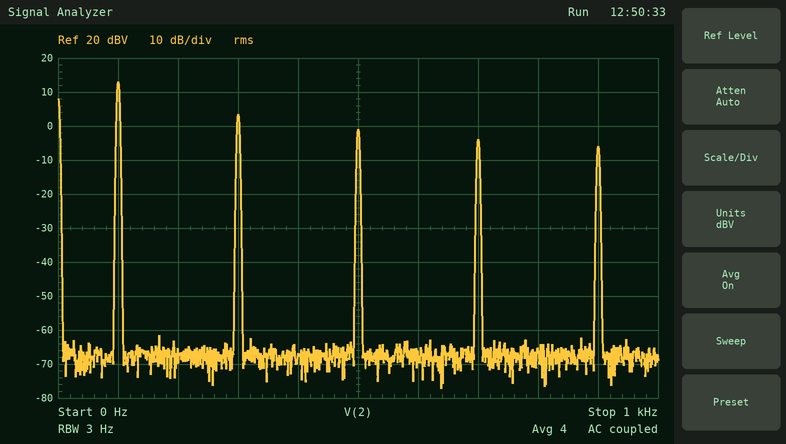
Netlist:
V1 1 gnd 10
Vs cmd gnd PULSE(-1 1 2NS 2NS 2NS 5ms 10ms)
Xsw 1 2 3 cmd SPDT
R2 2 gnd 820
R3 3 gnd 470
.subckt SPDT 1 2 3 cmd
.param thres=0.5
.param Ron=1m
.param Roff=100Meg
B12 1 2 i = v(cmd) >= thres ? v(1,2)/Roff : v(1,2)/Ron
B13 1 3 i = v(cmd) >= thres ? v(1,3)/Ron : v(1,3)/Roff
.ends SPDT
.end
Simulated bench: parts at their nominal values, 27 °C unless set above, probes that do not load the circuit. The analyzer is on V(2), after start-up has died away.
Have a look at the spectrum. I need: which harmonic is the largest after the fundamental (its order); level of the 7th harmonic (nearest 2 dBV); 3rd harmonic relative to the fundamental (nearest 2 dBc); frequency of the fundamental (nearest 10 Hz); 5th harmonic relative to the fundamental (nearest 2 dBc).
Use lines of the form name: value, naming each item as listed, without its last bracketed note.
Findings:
which harmonic is the largest after the fundamental: 3
level of the 7th harmonic: -4 dBV
3rd harmonic relative to the fundamental: -10 dBc
frequency of the fundamental: 100 Hz
5th harmonic relative to the fundamental: -14 dBc
